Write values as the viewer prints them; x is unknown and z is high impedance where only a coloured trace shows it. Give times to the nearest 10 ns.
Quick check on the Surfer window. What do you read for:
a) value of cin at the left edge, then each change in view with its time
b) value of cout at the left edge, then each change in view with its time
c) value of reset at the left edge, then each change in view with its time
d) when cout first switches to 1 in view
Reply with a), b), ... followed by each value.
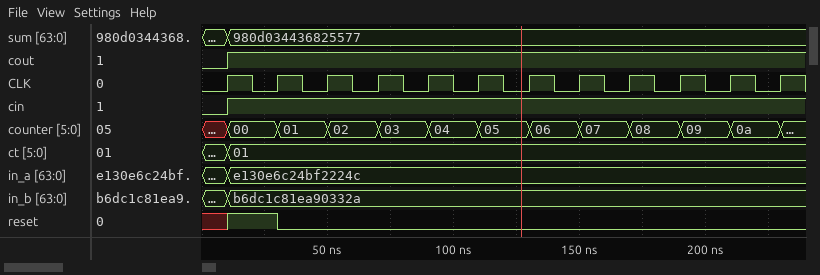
a) 0, 1 at 10 ns
b) 0, 1 at 10 ns
c) x, 1 at 10 ns, 0 at 30 ns
d) 10 ns
